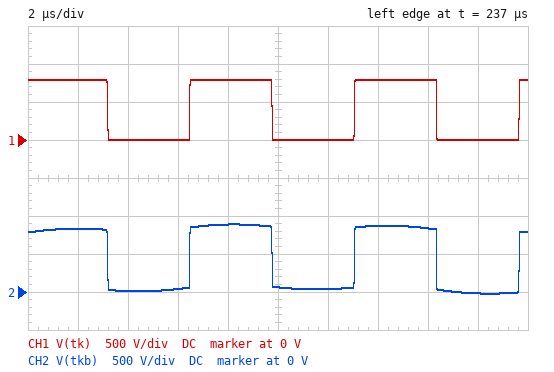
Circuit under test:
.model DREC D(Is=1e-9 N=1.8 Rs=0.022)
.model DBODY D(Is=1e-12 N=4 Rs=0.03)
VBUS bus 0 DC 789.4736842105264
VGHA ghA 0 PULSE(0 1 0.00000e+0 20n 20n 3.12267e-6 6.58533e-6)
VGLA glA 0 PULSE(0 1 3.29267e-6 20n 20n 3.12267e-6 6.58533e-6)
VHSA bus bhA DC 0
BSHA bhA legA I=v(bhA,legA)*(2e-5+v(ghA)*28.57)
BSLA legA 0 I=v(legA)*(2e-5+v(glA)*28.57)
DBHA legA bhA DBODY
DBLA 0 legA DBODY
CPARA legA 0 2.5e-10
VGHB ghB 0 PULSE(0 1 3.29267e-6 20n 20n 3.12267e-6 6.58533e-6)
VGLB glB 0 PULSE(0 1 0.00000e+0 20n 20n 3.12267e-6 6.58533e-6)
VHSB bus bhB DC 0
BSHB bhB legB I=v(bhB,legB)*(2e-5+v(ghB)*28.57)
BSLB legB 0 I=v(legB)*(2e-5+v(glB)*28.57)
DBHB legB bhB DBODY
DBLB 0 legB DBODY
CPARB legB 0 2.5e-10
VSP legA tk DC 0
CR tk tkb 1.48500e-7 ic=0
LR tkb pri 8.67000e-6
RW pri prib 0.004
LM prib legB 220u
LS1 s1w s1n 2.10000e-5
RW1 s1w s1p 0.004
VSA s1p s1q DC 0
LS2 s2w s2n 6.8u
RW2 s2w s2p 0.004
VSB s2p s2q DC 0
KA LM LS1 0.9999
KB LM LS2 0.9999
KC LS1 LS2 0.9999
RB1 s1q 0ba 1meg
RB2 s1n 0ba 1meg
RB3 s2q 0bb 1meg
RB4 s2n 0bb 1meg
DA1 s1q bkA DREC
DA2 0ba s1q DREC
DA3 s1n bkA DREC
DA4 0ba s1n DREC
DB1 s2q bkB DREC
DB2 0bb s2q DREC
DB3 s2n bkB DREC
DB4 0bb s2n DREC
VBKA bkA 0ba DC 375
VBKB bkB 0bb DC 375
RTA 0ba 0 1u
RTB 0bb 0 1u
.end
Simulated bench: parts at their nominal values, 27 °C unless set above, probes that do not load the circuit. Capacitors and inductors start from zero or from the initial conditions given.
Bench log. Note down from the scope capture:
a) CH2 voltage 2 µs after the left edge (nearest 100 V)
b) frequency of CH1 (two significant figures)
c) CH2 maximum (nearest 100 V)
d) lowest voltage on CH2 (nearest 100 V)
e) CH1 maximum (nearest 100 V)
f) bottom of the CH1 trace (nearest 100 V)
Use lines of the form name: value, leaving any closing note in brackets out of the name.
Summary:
CH2 voltage 2 µs after the left edge: 800 V
frequency of CH1: 150 kHz
CH2 maximum: 900 V
lowest voltage on CH2: 0 V
CH1 maximum: 800 V
bottom of the CH1 trace: 0 V
